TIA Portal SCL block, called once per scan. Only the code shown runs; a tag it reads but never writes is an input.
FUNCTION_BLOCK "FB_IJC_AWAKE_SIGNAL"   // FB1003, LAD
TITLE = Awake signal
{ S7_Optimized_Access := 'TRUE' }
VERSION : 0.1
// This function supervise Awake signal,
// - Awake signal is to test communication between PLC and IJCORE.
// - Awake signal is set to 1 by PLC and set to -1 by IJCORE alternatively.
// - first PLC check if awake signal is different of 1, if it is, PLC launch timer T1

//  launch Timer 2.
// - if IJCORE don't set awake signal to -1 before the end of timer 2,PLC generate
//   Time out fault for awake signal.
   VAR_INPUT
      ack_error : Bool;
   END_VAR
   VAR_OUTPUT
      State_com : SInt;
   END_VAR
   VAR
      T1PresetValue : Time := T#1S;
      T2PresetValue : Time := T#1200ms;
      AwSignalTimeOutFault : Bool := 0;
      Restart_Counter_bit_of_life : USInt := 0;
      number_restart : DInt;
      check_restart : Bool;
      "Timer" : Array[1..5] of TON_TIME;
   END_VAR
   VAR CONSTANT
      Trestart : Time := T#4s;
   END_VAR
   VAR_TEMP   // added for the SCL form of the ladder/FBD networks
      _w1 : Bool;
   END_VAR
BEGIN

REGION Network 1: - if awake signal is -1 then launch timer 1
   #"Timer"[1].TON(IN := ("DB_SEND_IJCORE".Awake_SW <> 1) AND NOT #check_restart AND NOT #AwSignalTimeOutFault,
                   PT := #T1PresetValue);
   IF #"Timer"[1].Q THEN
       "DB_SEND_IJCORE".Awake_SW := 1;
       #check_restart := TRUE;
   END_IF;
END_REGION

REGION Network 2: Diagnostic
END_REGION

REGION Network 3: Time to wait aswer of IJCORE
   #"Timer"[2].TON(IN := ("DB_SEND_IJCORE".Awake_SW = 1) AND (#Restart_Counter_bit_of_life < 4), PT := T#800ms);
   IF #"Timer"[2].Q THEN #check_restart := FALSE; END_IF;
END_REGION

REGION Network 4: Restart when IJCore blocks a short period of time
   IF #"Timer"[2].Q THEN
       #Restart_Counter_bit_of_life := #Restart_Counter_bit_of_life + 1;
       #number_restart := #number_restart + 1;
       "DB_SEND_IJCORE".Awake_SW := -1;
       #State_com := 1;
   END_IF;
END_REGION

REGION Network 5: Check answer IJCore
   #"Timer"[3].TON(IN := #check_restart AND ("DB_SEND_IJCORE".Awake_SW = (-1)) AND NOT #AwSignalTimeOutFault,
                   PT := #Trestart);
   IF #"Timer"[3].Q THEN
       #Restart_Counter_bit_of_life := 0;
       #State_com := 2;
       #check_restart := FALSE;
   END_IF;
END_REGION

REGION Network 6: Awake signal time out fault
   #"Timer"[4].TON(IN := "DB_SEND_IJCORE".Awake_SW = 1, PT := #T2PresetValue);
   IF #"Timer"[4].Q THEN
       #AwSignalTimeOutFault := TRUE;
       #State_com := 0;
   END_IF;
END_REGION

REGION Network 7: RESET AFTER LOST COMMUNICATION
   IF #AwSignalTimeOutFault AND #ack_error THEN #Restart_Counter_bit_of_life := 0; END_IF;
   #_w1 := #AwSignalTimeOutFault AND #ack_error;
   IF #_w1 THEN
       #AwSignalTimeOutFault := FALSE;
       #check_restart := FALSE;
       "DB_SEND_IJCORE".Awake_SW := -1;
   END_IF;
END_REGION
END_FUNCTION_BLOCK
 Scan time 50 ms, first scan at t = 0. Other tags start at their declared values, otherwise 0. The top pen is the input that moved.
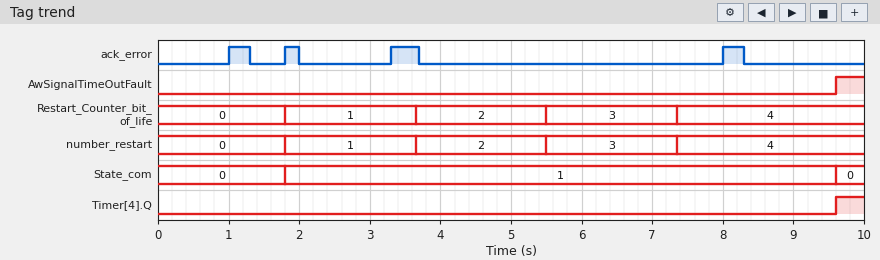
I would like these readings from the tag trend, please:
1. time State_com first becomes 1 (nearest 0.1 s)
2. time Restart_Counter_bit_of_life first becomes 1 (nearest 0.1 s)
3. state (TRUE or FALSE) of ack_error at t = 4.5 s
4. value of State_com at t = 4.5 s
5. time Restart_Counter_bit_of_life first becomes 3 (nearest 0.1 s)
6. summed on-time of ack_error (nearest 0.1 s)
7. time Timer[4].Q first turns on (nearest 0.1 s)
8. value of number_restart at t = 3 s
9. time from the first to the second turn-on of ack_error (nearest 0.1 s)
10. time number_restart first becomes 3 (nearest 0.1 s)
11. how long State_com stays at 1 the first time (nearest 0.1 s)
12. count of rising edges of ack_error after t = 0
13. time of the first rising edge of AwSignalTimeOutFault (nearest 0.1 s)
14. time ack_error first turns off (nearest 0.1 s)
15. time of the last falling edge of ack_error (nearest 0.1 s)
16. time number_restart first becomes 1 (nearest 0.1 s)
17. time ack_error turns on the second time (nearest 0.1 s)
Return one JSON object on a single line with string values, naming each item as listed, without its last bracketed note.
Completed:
{"time State_com first becomes 1": "1.8 s", "time Restart_Counter_bit_of_life first becomes 1": "1.8 s", "state (TRUE or FALSE) of ack_error at t = 4.5 s": "FALSE", "value of State_com at t = 4.5 s": "1", "time Restart_Counter_bit_of_life first becomes 3": "5.5 s", "summed on-time of ack_error": "1.2 s", "time Timer[4].Q first turns on": "9.6 s", "value of number_restart at t = 3 s": "1", "time from the first to the second turn-on of ack_error": "0.8 s", "time number_restart first becomes 3": "5.5 s", "how long State_com stays at 1 the first time": "7.8 s", "count of rising edges of ack_error after t = 0": "4", "time of the first rising edge of AwSignalTimeOutFault": "9.6 s", "time ack_error first turns off": "1.3 s", "time of the last falling edge of ack_error": "8.3 s", "time number_restart first becomes 1": "1.8 s", "time ack_error turns on the second time": "1.8 s"}
